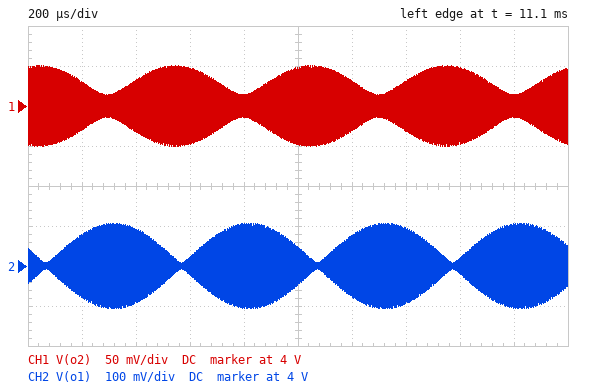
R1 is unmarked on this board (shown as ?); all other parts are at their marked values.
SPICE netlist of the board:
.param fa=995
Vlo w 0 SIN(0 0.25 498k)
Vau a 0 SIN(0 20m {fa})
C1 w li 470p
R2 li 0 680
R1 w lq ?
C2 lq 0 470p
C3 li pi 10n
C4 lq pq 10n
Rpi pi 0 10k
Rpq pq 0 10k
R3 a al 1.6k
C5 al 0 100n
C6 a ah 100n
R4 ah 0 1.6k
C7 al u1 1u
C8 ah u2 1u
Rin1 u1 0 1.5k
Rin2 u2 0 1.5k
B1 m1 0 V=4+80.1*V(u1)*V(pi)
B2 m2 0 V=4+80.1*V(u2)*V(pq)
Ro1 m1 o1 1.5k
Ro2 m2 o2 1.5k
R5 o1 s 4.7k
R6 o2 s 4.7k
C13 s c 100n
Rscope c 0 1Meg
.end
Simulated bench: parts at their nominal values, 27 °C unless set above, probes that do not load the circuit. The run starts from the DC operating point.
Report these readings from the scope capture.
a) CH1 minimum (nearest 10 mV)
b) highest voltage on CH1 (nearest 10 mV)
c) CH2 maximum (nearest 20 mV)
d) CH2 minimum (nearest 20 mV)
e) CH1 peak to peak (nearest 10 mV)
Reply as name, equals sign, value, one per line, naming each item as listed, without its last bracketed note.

CH1 minimum = 3.95 V
highest voltage on CH1 = 4.05 V
CH2 maximum = 4.10 V
CH2 minimum = 3.90 V
CH1 peak to peak = 100 mV
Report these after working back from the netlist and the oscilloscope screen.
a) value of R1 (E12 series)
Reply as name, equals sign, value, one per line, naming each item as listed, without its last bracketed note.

value of R1 = 1.8 kΩ
